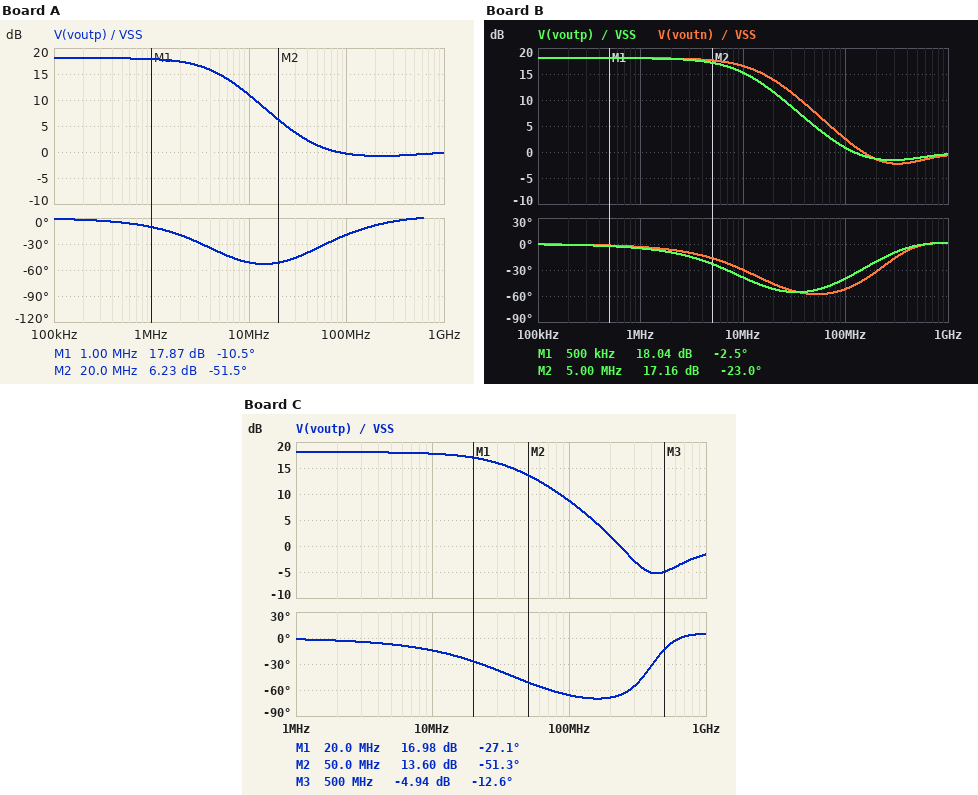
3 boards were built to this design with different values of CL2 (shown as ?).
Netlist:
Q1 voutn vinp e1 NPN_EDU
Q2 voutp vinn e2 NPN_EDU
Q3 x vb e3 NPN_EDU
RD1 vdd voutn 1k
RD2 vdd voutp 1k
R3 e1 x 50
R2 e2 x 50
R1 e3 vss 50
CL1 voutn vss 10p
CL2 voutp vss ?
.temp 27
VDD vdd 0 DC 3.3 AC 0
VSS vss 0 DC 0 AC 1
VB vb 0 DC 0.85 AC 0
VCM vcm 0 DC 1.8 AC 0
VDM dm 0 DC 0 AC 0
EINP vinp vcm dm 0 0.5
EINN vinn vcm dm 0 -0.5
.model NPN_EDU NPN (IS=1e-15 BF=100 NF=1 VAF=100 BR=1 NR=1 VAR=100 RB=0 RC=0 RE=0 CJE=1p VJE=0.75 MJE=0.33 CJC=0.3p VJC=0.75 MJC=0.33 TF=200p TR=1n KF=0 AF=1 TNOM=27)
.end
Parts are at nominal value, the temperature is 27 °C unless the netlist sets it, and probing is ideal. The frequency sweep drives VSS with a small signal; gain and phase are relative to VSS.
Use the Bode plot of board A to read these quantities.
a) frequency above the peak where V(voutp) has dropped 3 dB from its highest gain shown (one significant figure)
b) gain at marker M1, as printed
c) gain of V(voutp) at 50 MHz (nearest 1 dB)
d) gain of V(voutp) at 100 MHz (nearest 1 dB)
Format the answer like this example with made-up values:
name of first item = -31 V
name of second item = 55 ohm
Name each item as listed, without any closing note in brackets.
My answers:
frequency above the peak where V(voutp) has dropped 3 dB from its highest gain shown = 5 MHz
gain at marker M1, as printed = 17.87 dB
gain of V(voutp) at 50 MHz = 1 dB
gain of V(voutp) at 100 MHz = 0 dB
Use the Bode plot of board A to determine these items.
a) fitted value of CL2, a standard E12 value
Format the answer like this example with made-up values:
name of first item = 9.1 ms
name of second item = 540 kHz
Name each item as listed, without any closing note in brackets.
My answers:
fitted value of CL2, a standard E12 value = 33 pF
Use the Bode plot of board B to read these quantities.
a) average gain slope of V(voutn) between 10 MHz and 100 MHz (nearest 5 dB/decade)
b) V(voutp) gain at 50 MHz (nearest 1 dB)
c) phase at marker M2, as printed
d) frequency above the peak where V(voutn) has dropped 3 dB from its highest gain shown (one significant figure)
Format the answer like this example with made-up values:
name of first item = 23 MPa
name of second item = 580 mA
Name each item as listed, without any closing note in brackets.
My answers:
average gain slope of V(voutn) between 10 MHz and 100 MHz = -15 dB/decade
V(voutp) gain at 50 MHz = 5 dB
phase at marker M2, as printed = -23.0 deg
frequency above the peak where V(voutn) has dropped 3 dB from its highest gain shown = 20 MHz
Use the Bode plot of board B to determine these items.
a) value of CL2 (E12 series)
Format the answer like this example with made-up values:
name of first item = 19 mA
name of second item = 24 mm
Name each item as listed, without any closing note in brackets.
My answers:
value of CL2 = 15 pF
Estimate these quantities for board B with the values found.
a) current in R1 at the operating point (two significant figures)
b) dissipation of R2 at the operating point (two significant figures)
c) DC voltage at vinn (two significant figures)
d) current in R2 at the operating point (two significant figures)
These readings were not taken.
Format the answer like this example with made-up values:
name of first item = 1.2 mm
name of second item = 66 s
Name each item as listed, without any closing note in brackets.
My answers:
current in R1 at the operating point = 2.3 mA
dissipation of R2 at the operating point = 64 µW
DC voltage at vinn = 1.8 V
current in R2 at the operating point = 1.1 mA
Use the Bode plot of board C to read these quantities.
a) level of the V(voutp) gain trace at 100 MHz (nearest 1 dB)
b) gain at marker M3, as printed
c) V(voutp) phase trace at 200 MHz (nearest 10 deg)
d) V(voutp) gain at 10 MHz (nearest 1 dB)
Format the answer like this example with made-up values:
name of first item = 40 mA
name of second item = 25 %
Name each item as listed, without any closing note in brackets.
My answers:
level of the V(voutp) gain trace at 100 MHz = 9 dB
gain at marker M3, as printed = -4.94 dB
V(voutp) phase trace at 200 MHz = -70 deg
V(voutp) gain at 10 MHz = 18 dB
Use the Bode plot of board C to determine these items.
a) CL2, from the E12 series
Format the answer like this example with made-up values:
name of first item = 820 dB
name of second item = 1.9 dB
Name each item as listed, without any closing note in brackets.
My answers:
CL2, from the E12 series = 3.9 pF
